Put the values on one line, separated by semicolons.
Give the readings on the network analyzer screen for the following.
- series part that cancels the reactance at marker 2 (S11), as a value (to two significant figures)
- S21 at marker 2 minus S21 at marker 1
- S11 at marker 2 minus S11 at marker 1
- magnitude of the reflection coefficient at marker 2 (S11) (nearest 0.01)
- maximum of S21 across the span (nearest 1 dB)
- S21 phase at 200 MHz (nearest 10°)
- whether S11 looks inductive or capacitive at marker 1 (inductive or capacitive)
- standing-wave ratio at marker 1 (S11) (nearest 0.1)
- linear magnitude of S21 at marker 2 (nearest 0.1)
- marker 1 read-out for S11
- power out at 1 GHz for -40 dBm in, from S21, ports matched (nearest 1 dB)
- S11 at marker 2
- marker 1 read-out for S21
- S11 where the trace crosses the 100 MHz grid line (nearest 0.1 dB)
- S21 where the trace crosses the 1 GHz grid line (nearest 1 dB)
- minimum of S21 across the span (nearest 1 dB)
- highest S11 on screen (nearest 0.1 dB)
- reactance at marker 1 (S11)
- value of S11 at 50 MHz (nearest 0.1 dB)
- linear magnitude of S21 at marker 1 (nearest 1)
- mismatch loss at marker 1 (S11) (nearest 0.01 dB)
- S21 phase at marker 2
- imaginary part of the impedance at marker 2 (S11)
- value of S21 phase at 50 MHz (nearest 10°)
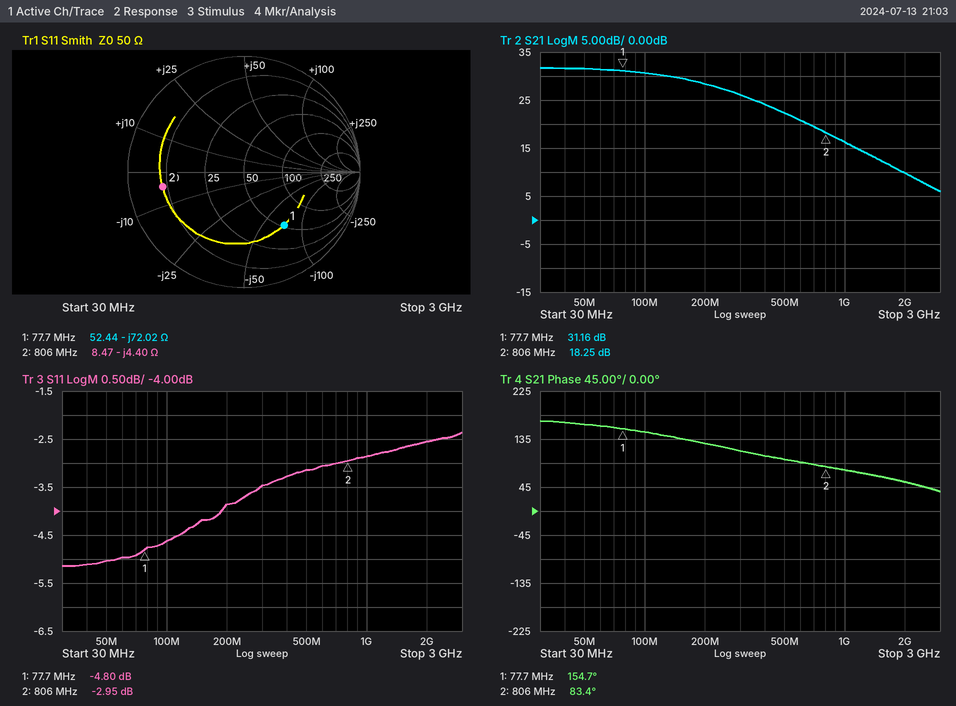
870 pH; -12.91 dB; 1.85 dB; 0.71; 32 dB; 130°; capacitive; 3.7; 8.2; -4.80 dB; -24 dBm; -2.95 dB; 31.16 dB; -4.6 dB; 16 dB; 6 dB; -2.4 dB; -72.02 Ω; -5.0 dB; 36; 1.75 dB; 83.4°; -4.40 Ω; 160°
